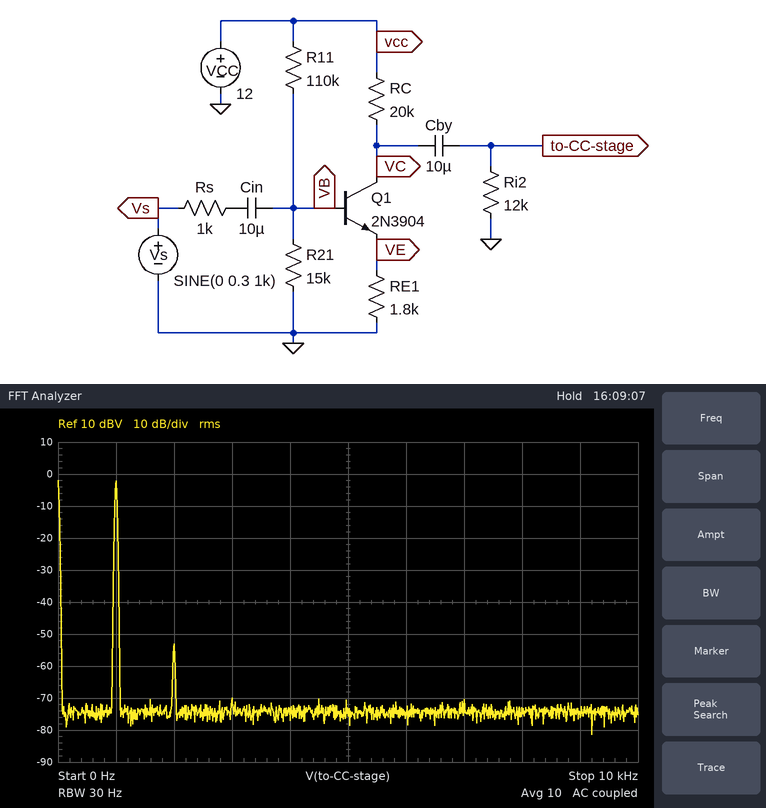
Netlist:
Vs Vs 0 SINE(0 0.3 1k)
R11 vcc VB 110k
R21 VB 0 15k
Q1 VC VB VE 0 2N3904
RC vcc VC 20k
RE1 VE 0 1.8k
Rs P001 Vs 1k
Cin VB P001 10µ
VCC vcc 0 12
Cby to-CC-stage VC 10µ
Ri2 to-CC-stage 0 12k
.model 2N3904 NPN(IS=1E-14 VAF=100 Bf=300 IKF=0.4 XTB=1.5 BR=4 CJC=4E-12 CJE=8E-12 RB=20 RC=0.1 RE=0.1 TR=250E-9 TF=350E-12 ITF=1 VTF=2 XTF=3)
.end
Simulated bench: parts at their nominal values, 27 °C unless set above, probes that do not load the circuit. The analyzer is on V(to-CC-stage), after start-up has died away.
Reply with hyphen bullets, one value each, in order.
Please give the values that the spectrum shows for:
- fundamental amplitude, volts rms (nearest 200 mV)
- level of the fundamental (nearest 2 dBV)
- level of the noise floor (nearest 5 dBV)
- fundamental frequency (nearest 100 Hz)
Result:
- 800 mV
- -2 dBV
- -75 dBV
- 1.0 kHz
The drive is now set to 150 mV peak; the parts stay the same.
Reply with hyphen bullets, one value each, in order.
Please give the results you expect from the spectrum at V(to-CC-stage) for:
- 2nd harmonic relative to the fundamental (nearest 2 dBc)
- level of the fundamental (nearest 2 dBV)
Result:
- -58 dBc
- -8 dBV
